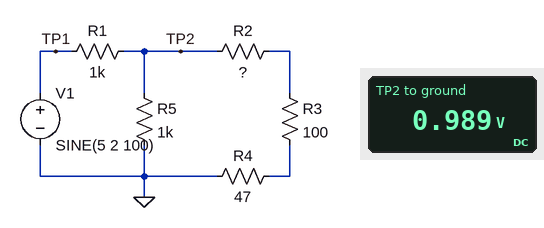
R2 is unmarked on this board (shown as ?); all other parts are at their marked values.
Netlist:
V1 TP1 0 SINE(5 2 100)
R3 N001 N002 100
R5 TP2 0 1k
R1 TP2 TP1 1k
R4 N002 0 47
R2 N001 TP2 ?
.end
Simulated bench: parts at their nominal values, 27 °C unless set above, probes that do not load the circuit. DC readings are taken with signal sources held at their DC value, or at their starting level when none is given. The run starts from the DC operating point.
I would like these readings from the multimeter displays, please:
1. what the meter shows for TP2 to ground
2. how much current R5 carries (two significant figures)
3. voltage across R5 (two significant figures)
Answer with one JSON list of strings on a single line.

["0.989 V", "990 µA", "990 mV"]
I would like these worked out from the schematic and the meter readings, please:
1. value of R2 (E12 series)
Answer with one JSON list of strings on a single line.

["180 Ω"]
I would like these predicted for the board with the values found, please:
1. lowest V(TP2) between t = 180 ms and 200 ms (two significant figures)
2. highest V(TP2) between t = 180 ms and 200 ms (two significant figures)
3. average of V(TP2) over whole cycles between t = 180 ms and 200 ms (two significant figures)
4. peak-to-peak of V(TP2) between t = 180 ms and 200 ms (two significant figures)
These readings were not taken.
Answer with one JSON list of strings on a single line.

["590 mV", "1.4 V", "990 mV", "790 mV"]
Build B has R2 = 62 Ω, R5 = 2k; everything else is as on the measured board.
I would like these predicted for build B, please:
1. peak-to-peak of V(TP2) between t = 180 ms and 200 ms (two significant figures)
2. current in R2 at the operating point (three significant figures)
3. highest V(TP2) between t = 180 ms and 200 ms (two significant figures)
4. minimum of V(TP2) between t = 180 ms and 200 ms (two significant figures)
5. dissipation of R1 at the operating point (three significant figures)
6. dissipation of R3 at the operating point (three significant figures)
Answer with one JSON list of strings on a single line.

["640 mV", "3.81 mA", "1.1 V", "480 mV", "17.7 mW", "1.45 mW"]
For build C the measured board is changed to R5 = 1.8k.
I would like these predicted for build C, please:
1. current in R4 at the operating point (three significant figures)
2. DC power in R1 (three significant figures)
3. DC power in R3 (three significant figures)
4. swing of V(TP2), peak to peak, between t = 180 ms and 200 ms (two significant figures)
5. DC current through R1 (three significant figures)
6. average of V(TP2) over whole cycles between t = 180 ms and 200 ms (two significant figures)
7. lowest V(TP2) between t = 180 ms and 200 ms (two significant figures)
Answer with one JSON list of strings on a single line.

["3.31 mA", "15.3 mW", "1.10 mW", "870 mV", "3.92 mA", "1.1 V", "650 mV"]
